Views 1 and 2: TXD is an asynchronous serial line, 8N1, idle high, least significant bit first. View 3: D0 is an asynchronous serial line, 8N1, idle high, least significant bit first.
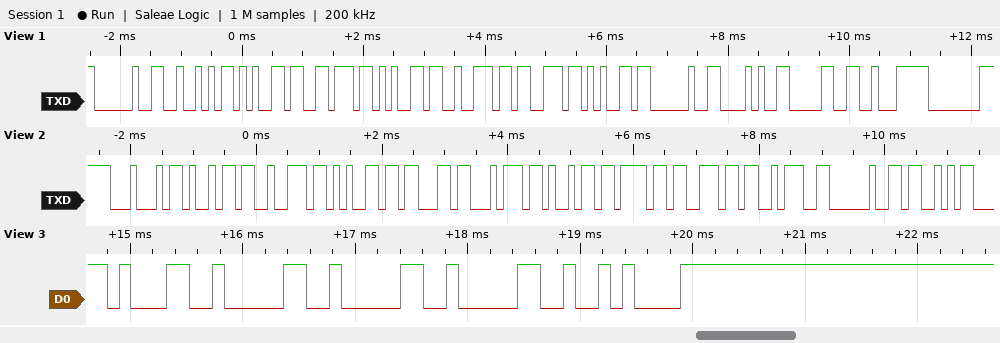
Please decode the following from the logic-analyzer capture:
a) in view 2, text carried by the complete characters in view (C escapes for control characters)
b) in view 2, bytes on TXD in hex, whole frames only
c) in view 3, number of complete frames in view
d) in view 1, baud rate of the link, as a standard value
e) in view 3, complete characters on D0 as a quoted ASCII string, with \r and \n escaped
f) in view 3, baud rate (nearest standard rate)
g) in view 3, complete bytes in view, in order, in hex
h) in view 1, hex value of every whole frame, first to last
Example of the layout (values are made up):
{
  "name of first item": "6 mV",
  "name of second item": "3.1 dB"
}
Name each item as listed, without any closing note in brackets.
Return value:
{
  "in view 2, text carried by the complete characters in view": "\"Direction: S\"",
  "in view 2, bytes on TXD in hex, whole frames only": "0x44 0x69 0x72 0x65 0x63 0x74 0x69 0x6F 0x6E 0x3A 0x20 0x53",
  "in view 3, number of complete frames in view": "5",
  "in view 1, baud rate of the link, as a standard value": "9600 baud",
  "in view 3, complete characters on D0 as a quoted ASCII string, with \\r and \\n escaped": "\"1000\\n\"",
  "in view 3, baud rate": "9600 baud",
  "in view 3, complete bytes in view, in order, in hex": "31 30 30 30 0A",
  "in view 1, hex value of every whole frame, first to last": "20 52 65 76 65 72 73 65 20 28 30 E2 80"
}
